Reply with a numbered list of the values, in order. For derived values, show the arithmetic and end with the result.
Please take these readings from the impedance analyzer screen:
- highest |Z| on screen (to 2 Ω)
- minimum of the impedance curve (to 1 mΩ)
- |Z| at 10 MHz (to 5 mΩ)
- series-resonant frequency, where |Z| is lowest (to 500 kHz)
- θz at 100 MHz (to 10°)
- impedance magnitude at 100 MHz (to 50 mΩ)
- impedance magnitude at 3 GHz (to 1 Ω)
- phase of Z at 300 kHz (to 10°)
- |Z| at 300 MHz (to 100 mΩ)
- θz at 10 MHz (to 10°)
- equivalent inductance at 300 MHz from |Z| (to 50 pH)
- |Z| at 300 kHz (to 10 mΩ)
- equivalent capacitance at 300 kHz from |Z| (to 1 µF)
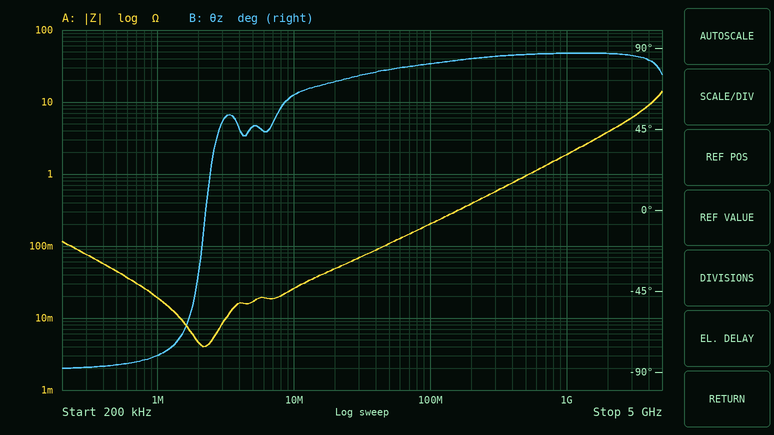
1. 14 Ω
2. 4 mΩ
3. 25 mΩ
4. 2.0 MHz
5. 80°
6. 200 mΩ
7. 6 Ω
8. -90°
9. 600 mΩ
10. 60°
11. L = 600 mΩ/(2π × 300 MHz) ≈ 318 pH, so 300 pH to the nearest 50 pH
12. 80 mΩ
13. C = 1/(2π × 300 kHz × 80 mΩ) ≈ 7 µF
